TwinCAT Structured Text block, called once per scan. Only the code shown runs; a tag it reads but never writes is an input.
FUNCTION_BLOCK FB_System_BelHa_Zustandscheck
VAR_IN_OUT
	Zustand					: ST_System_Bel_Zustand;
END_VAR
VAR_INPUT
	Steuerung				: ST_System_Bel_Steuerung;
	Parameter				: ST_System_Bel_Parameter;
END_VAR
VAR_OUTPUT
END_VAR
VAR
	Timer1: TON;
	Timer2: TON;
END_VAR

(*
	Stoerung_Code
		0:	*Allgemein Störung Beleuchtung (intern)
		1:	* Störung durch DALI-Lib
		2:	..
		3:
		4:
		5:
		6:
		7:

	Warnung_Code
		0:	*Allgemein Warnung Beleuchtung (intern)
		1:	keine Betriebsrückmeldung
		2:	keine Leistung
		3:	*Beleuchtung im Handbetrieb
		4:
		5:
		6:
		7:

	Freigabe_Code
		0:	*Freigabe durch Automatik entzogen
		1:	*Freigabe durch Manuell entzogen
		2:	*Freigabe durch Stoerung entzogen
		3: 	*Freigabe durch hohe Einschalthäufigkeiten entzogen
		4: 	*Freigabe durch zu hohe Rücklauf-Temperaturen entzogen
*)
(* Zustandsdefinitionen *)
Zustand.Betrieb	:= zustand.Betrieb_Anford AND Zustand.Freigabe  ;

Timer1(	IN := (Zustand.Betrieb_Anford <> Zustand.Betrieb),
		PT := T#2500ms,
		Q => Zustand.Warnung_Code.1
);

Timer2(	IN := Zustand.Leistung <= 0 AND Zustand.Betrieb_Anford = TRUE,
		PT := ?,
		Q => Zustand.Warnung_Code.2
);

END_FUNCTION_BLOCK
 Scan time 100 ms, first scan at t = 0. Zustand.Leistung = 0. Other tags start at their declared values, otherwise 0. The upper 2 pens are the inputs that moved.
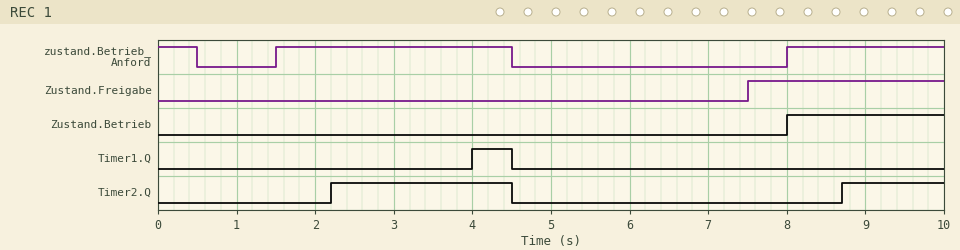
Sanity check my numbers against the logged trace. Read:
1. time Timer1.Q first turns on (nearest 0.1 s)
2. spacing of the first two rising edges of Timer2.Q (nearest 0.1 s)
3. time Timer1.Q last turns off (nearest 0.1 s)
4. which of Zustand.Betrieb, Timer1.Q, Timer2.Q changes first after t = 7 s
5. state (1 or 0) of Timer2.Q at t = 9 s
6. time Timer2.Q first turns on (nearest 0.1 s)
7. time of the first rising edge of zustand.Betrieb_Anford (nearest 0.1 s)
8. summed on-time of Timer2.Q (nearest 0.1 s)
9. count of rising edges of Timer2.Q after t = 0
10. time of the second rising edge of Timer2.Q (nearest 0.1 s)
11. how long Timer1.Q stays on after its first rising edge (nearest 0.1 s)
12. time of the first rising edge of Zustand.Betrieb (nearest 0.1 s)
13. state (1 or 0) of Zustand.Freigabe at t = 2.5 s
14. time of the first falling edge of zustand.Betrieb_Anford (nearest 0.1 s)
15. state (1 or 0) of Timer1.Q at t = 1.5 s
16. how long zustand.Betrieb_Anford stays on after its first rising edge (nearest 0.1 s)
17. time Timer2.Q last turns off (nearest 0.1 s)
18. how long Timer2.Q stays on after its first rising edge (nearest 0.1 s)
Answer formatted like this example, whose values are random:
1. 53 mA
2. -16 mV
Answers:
1. 4.0 s
2. 6.5 s
3. 4.5 s
4. Zustand.Betrieb
5. 1
6. 2.2 s
7. 1.5 s
8. 3.6 s
9. 2
10. 8.7 s
11. 0.5 s
12. 8.0 s
13. 0
14. 0.5 s
15. 0
16. 3.0 s
17. 4.5 s
18. 2.3 s
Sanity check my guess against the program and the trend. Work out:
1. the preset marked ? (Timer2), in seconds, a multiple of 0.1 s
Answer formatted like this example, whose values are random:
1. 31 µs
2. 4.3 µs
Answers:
1. 0.7 s
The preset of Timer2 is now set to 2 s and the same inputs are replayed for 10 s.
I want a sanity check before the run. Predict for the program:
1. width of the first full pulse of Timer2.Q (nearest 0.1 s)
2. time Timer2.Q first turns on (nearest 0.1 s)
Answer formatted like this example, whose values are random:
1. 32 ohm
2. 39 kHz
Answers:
1. 1.0 s
2. 3.5 s
